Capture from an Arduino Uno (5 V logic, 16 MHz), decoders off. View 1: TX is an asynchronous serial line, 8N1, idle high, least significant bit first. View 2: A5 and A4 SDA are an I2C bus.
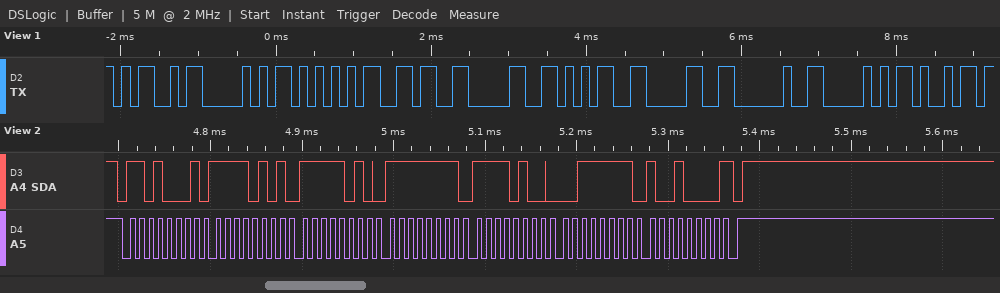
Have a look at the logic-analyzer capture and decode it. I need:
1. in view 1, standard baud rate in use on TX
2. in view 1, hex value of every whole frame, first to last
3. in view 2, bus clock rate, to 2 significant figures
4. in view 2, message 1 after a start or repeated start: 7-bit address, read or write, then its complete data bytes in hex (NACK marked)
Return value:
9600 baud
0x4D 0x50 0x55 0x36 0x30 0x35 0x30 0x20 0x50 0x69
100 kHz
0x68 read: F5 FA FF F4 3F 90 NACK
